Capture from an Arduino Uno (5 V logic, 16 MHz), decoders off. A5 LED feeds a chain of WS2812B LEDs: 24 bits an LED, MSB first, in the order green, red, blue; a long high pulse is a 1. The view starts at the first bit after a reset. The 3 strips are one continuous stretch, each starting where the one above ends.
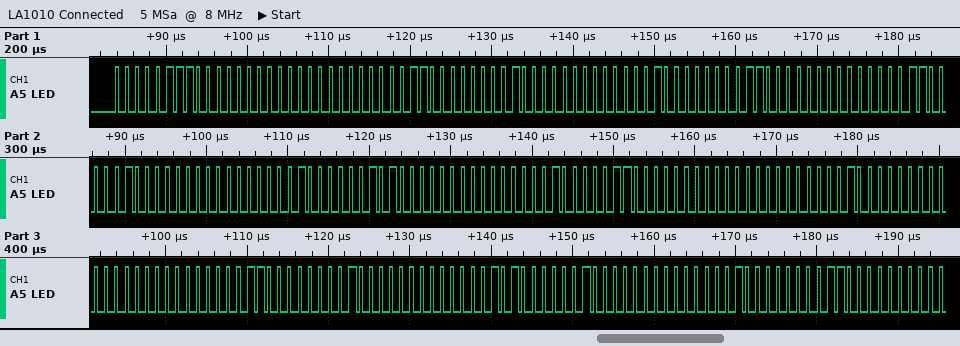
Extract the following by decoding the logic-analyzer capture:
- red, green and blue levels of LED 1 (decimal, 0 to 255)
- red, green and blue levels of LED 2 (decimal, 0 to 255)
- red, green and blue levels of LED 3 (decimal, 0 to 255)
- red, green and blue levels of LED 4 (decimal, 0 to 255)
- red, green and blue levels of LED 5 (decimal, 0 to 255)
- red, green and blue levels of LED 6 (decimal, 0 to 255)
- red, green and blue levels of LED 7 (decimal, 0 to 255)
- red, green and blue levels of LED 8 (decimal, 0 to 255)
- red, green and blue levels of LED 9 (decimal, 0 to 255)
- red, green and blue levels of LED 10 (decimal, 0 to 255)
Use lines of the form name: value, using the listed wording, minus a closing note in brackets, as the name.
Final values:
red, green and blue levels of LED 1: 0, 7, 0
red, green and blue levels of LED 2: 1, 6, 0
red, green and blue levels of LED 3: 3, 4, 0
red, green and blue levels of LED 4: 4, 3, 0
red, green and blue levels of LED 5: 5, 2, 0
red, green and blue levels of LED 6: 6, 1, 0
red, green and blue levels of LED 7: 8, 0, 0
red, green and blue levels of LED 8: 6, 0, 1
red, green and blue levels of LED 9: 5, 0, 2
red, green and blue levels of LED 10: 4, 0, 3
